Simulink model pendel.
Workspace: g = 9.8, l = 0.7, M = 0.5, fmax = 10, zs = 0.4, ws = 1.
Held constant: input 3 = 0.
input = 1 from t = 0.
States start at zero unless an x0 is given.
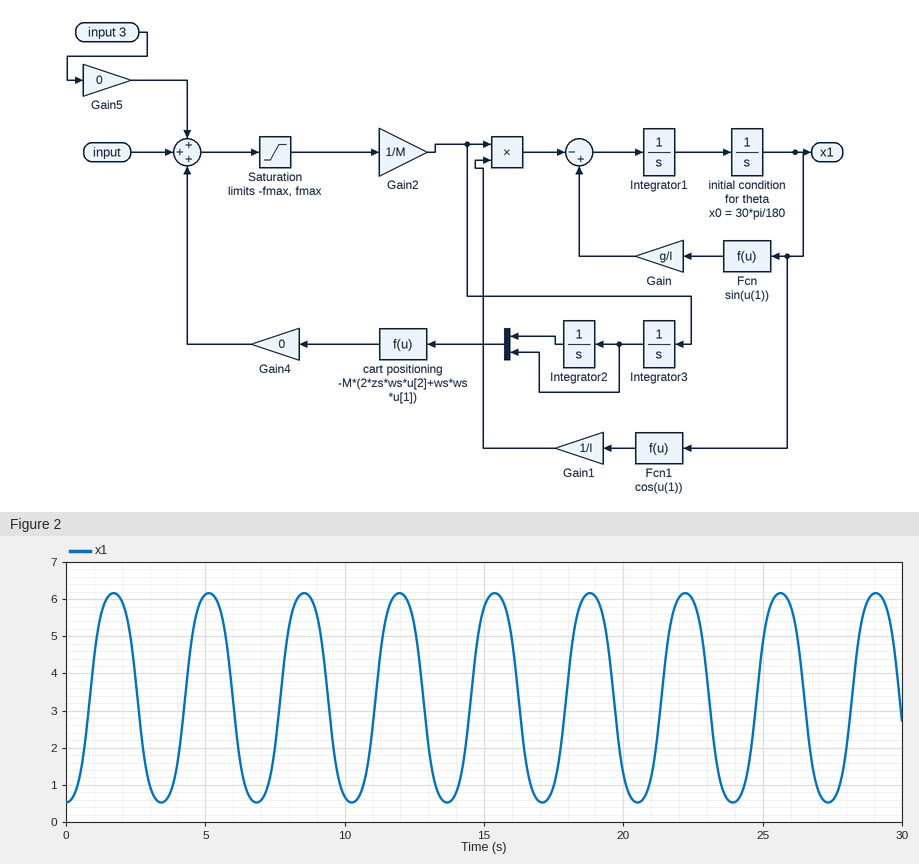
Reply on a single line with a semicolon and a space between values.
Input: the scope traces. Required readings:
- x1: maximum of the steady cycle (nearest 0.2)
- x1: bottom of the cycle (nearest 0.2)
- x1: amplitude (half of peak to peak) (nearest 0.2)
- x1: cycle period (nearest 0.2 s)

6.2; 0.6; 2.8; 3.4 s
